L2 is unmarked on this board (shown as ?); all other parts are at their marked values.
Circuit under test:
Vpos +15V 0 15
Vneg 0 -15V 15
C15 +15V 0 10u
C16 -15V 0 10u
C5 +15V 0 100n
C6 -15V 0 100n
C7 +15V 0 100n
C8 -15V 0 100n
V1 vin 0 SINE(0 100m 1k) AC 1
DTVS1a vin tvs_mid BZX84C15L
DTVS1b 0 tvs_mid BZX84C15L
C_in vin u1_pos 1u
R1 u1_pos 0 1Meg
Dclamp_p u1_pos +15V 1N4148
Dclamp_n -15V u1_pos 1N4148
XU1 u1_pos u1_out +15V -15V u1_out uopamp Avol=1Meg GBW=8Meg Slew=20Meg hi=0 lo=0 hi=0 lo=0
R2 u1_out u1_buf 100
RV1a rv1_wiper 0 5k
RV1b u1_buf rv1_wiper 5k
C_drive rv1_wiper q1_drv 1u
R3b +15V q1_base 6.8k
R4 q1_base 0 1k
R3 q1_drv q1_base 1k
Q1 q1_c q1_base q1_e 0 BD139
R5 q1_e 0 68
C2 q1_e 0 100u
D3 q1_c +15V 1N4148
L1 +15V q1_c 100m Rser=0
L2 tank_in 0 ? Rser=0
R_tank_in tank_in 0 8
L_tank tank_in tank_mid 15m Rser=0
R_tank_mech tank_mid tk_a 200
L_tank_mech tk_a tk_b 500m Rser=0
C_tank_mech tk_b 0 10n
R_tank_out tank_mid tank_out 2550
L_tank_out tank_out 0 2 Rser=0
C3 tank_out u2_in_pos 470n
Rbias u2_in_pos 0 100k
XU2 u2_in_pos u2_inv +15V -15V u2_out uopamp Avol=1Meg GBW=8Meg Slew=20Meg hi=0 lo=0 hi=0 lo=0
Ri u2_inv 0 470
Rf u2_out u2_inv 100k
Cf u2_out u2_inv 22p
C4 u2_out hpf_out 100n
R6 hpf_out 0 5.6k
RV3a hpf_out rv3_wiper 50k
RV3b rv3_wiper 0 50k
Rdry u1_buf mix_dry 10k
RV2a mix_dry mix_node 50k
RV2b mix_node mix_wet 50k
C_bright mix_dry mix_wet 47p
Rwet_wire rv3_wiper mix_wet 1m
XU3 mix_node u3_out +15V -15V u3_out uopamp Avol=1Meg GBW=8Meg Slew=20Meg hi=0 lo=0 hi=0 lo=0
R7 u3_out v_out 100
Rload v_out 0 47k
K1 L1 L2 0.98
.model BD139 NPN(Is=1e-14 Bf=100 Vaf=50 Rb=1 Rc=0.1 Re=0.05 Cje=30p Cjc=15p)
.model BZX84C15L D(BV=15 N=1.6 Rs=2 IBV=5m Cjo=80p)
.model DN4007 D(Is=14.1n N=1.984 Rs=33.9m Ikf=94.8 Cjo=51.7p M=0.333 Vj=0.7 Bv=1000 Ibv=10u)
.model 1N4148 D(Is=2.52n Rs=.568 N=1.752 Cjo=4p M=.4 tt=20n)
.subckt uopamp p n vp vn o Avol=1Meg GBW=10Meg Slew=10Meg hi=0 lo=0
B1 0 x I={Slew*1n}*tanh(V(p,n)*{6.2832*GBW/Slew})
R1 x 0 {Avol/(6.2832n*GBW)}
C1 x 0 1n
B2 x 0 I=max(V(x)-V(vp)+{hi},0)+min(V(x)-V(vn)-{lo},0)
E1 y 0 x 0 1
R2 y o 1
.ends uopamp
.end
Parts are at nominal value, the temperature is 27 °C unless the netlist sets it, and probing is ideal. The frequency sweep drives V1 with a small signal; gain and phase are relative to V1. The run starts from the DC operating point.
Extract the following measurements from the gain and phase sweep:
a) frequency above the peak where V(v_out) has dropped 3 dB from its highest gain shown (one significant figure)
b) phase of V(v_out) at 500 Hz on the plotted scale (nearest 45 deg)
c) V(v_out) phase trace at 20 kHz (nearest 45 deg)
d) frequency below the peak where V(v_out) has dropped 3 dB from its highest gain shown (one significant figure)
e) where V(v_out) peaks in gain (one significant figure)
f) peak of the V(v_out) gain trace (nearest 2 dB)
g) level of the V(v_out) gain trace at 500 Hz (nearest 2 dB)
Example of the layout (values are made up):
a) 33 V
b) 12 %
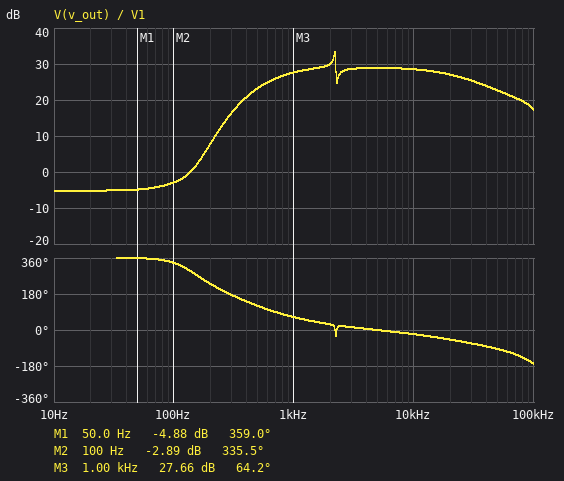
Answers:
a) 2 kHz
b) 135 deg
c) -45 deg
d) 2 kHz
e) 2 kHz
f) 34 dB
g) 24 dB
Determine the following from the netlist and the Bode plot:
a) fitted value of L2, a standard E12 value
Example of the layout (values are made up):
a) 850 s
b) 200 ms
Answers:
a) 2.7 mH
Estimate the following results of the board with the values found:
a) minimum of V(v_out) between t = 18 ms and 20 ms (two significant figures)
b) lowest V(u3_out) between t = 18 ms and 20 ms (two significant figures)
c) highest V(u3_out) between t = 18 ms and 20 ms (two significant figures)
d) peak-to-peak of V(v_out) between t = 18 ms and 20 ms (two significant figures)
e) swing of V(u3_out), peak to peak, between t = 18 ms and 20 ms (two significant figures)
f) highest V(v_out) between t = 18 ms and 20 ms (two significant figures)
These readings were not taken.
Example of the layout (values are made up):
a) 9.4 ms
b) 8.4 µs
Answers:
a) -2.4 V
b) -2.4 V
c) 2.4 V
d) 4.8 V
e) 4.8 V
f) 2.4 V
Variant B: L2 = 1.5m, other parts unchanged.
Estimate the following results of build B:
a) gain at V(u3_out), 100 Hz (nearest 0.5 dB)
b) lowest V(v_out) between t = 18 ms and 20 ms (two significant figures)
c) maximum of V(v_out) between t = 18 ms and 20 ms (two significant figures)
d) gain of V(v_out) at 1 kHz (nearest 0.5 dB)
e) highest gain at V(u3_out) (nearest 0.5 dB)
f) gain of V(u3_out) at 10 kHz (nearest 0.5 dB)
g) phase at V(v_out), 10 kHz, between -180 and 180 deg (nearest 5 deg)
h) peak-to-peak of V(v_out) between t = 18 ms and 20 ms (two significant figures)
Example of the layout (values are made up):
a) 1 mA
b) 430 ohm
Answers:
a) -3.5 dB
b) -2.6 V
c) 2.7 V
d) 28.5 dB
e) 35.5 dB
f) 30.5 dB
g) -20 deg
h) 5.2 V
